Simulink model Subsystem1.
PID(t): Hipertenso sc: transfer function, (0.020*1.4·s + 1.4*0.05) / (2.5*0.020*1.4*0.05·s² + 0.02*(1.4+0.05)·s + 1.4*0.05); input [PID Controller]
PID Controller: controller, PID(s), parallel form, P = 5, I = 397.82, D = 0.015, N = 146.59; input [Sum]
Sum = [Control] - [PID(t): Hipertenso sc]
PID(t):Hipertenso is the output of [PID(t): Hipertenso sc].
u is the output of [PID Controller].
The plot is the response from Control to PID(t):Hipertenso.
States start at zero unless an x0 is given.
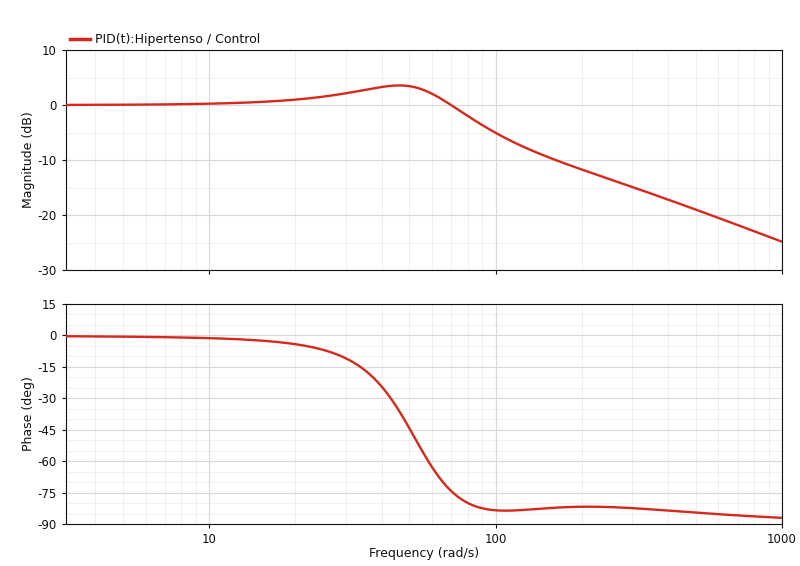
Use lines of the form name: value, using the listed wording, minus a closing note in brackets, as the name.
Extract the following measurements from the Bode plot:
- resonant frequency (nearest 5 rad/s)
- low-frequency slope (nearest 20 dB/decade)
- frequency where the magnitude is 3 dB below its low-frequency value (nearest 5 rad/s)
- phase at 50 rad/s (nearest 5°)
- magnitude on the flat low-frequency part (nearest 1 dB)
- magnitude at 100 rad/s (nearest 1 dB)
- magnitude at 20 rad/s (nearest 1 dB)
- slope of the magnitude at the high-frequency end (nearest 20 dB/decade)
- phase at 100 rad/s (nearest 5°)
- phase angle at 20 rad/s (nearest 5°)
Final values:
resonant frequency: 45 rad/s
low-frequency slope: 0 dB/decade
frequency where the magnitude is 3 dB below its low-frequency value: 85 rad/s
phase at 50 rad/s: -45°
magnitude on the flat low-frequency part: 0 dB
magnitude at 100 rad/s: -5 dB
magnitude at 20 rad/s: 1 dB
slope of the magnitude at the high-frequency end: -20 dB/decade
phase at 100 rad/s: -85°
phase angle at 20 rad/s: -5°
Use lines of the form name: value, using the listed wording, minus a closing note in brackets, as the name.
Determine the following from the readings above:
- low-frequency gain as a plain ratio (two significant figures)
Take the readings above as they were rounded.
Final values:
low-frequency gain as a plain ratio: 1.0
